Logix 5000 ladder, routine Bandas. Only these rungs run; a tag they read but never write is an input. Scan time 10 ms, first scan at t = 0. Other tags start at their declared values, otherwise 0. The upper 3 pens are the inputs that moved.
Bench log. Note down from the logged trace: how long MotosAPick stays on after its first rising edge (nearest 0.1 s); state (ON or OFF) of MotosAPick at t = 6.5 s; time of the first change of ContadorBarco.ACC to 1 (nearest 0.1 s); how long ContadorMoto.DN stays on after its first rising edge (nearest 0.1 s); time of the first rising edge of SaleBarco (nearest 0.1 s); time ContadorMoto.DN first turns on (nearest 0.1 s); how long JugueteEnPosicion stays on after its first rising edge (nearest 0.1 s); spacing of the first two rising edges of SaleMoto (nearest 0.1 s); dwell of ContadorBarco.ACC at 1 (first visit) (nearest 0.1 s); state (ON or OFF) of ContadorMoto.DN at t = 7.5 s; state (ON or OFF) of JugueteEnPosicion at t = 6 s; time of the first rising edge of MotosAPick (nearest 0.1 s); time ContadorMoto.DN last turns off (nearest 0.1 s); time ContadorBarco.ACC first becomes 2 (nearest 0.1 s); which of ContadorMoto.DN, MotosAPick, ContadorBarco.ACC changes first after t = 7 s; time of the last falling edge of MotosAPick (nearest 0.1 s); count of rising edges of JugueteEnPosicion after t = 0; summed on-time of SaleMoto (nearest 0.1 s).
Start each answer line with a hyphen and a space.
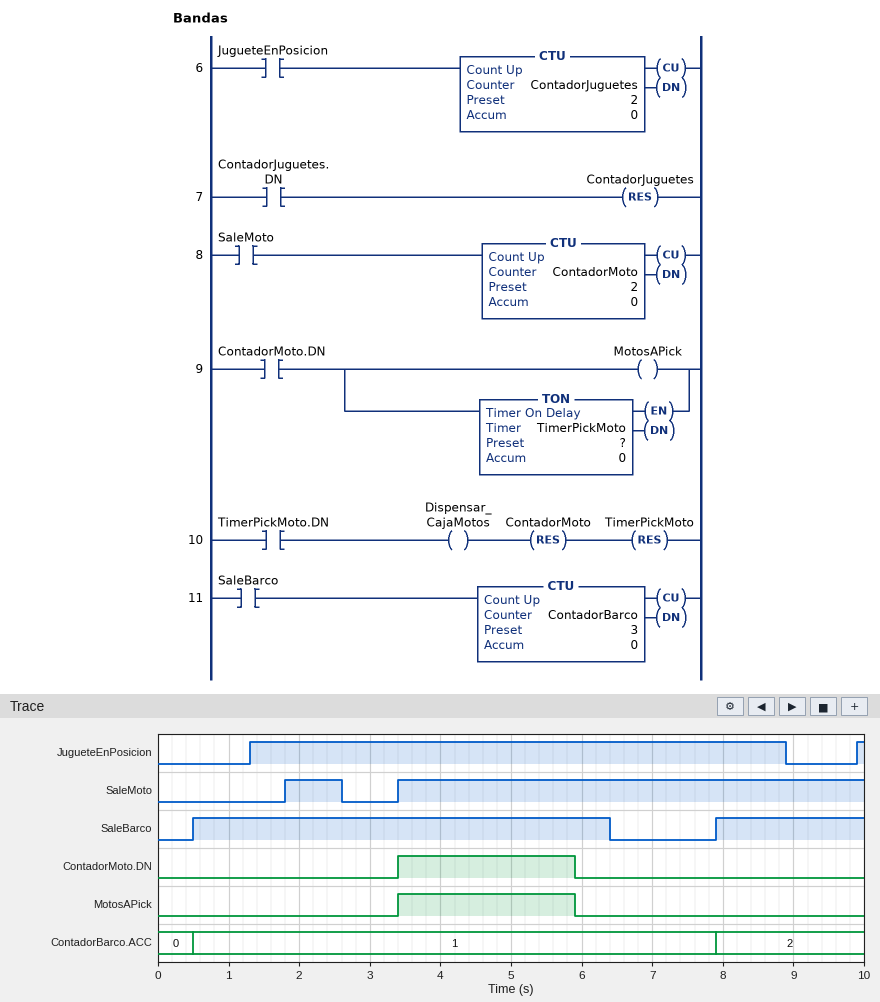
- 2.5 s
- OFF
- 0.5 s
- 2.5 s
- 0.5 s
- 3.4 s
- 7.6 s
- 1.6 s
- 7.4 s
- OFF
- ON
- 3.4 s
- 5.9 s
- 7.9 s
- ContadorBarco.ACC
- 5.9 s
- 2
- 7.4 s
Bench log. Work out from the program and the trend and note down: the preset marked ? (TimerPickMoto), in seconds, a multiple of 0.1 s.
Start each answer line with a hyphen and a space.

- 2.5 s
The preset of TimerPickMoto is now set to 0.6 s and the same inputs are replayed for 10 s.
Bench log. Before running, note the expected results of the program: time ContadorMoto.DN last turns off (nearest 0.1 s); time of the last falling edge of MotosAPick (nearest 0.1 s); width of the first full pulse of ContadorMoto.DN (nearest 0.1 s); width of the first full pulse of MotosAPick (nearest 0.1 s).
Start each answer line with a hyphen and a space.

- 4.0 s
- 4.0 s
- 0.6 s
- 0.6 s
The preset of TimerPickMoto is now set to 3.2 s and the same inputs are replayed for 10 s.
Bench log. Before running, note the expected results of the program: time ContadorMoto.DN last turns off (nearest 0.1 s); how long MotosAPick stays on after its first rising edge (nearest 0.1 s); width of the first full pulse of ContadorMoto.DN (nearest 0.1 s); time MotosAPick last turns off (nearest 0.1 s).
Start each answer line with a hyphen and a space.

- 6.6 s
- 3.2 s
- 3.2 s
- 6.6 s
